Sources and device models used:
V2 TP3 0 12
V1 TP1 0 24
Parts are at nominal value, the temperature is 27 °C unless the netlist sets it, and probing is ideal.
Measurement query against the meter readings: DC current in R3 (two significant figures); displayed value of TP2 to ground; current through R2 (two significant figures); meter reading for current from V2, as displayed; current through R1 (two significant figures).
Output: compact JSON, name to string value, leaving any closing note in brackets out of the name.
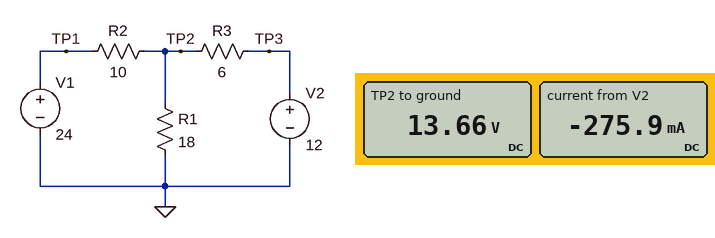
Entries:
{"DC current in R3": "280 mA", "displayed value of TP2 to ground": "13.66 V", "current through R2": "1.0 A", "meter reading for current from V2, as displayed": "-275.9 mA", "current through R1": "760 mA"}
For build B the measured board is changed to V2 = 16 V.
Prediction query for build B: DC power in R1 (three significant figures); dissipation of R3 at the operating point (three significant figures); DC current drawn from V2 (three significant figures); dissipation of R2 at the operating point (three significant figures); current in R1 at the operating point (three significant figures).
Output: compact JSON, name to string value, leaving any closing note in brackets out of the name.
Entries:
{"DC power in R1": "13.7 W", "dissipation of R3 at the operating point": "12.7 mW", "DC current drawn from V2": "46.0 mA", "dissipation of R2 at the operating point": "6.85 W", "current in R1 at the operating point": "874 mA"}
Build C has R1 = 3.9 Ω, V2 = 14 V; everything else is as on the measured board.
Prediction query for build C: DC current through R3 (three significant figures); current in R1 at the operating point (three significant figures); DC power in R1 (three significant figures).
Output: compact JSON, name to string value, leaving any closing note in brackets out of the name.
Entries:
{"DC current through R3": "825 mA", "current in R1 at the operating point": "2.32 A", "DC power in R1": "21.0 W"}
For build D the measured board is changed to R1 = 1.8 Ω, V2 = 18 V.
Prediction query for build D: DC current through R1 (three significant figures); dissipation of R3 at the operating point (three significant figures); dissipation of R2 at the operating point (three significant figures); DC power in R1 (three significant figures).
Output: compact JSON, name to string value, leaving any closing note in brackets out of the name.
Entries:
{"DC current through R1": "3.65 A", "dissipation of R3 at the operating point": "21.8 W", "dissipation of R2 at the operating point": "30.4 W", "DC power in R1": "24.0 W"}
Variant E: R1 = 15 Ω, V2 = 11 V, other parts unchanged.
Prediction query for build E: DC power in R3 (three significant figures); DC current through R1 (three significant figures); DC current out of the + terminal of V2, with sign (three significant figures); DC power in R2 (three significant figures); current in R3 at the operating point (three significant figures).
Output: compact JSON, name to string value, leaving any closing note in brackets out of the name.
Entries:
{"DC power in R3": "482 mW", "DC current through R1": "847 mA", "DC current out of the + terminal of V2, with sign": "-283 mA", "DC power in R2": "12.8 W", "current in R3 at the operating point": "283 mA"}
